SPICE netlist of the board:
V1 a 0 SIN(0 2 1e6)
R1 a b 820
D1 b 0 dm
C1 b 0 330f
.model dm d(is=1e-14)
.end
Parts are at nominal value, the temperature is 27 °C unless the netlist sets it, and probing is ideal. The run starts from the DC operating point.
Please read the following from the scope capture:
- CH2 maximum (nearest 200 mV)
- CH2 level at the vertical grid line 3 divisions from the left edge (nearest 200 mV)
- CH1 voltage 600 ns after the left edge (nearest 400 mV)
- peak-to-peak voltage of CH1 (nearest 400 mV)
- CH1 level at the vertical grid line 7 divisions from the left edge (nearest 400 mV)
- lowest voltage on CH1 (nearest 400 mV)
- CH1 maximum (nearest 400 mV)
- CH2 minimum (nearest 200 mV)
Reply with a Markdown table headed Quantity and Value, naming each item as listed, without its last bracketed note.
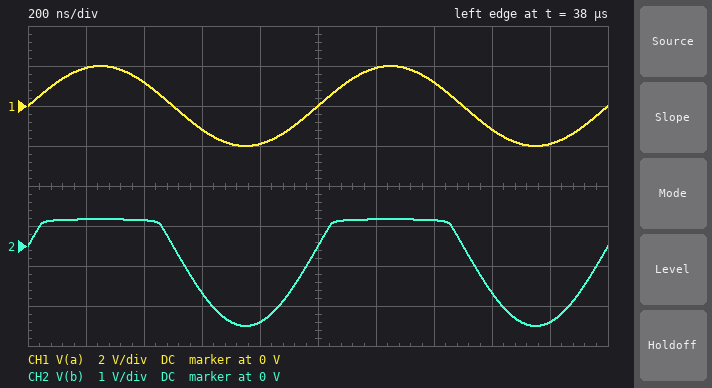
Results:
| Quantity | Value |
|---|---|
| CH2 maximum | 600 mV |
| CH2 level at the vertical grid line 3 divisions from the left edge | -1.2 V |
| CH1 voltage 600 ns after the left edge | -1.2 V |
| peak-to-peak voltage of CH1 | 4.0 V |
| CH1 level at the vertical grid line 7 divisions from the left edge | 1.2 V |
| lowest voltage on CH1 | -2.0 V |
| CH1 maximum | 2.0 V |
| CH2 minimum | -2.0 V |
